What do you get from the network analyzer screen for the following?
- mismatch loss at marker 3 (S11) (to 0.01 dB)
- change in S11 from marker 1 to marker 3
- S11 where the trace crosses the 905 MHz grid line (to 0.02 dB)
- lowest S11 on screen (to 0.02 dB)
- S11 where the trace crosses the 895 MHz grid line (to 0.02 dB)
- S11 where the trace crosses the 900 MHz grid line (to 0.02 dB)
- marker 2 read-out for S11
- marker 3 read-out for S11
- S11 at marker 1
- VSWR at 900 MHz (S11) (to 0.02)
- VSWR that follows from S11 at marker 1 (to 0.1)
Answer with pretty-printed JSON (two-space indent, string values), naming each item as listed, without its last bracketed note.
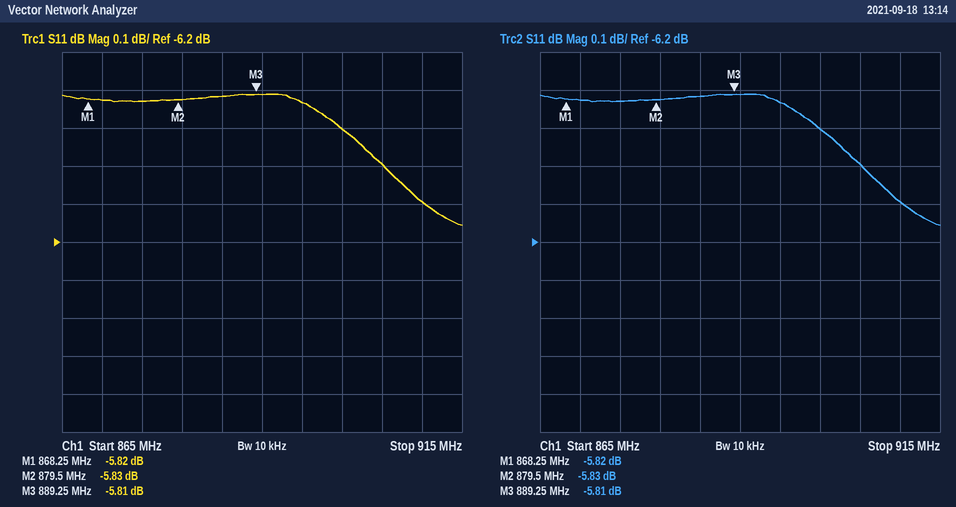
{
  "mismatch loss at marker 3 (S11)": "1.32 dB",
  "change in S11 from marker 1 to marker 3": "0.01 dB",
  "S11 where the trace crosses the 905 MHz grid line": "-6.00 dB",
  "lowest S11 on screen": "-6.16 dB",
  "S11 where the trace crosses the 895 MHz grid line": "-5.84 dB",
  "S11 where the trace crosses the 900 MHz grid line": "-5.90 dB",
  "marker 2 read-out for S11": "-5.83 dB",
  "marker 3 read-out for S11": "-5.81 dB",
  "S11 at marker 1": "-5.82 dB",
  "VSWR at 900 MHz (S11)": "3.06",
  "VSWR that follows from S11 at marker 1": "3.1"
}
